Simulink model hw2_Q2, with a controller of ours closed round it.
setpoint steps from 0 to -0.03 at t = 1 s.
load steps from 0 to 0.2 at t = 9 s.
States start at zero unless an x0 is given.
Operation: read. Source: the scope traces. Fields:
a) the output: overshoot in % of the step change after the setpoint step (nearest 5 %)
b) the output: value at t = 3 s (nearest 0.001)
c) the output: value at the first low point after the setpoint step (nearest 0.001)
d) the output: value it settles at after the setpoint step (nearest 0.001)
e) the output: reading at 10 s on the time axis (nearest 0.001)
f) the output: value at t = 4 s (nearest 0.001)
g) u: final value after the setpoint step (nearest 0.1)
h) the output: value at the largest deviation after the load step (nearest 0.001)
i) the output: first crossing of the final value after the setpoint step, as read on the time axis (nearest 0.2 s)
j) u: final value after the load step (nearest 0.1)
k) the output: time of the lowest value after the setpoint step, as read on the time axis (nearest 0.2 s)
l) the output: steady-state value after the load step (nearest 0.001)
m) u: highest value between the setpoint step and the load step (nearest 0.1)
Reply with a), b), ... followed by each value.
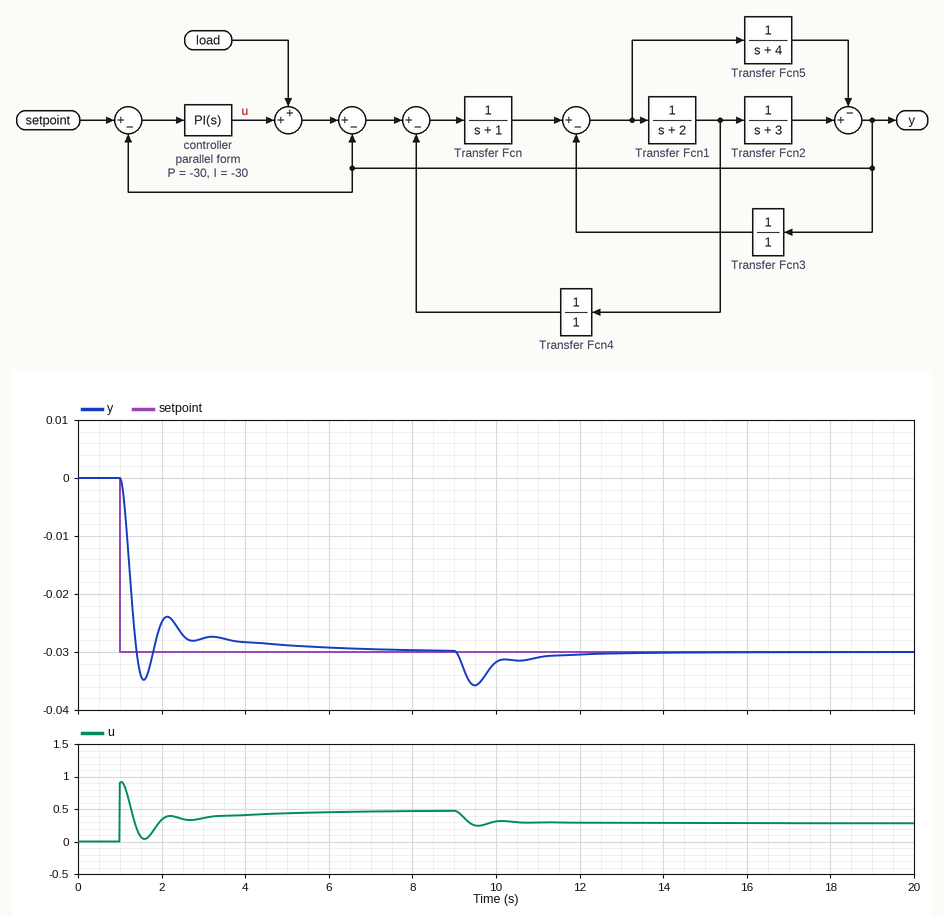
a) 15 %
b) -0.028
c) -0.035
d) -0.030
e) -0.032
f) -0.028
g) 0.5
h) -0.036
i) 1.4 s
j) 0.3
k) 1.6 s
l) -0.030
m) 0.9
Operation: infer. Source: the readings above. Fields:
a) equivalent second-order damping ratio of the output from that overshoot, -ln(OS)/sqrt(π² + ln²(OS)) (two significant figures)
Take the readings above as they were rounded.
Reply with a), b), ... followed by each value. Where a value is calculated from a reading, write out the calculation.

a) ln(0.15) = -1.897; 1.897 / sqrt(9.870 + 3.599) = 0.52
